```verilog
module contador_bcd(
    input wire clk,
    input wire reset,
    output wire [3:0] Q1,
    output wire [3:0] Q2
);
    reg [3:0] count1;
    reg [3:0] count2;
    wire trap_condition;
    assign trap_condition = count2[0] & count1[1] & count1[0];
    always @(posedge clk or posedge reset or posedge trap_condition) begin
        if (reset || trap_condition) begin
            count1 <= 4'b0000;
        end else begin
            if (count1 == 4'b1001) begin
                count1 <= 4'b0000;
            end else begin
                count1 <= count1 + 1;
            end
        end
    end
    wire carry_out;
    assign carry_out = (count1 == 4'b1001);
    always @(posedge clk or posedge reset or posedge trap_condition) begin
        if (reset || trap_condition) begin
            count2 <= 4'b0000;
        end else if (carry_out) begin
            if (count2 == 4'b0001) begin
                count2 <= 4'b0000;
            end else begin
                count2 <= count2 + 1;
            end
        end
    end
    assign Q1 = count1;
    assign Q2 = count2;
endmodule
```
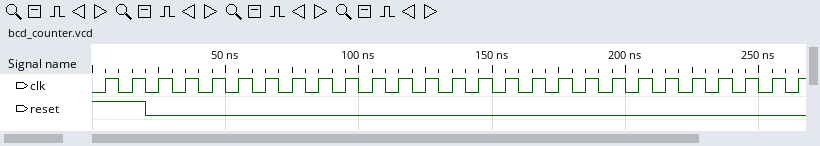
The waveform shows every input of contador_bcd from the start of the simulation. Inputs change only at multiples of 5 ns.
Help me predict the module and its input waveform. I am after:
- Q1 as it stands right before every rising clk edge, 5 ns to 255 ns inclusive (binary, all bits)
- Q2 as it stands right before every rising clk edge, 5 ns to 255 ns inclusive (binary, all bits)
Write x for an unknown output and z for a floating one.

0000, 0000, 0000, 0001, 0010, 0011, 0100, 0101, 0110, 0111, 1000, 1001, 0000, 0001, 0010, 0000, 0001, 0010, 0011, 0100, 0101, 0110, 0111, 1000, 1001, 0000
0000, 0000, 0000, 0000, 0000, 0000, 0000, 0000, 0000, 0000, 0000, 0000, 0001, 0001, 0001, 0000, 0000, 0000, 0000, 0000, 0000, 0000, 0000, 0000, 0000, 0001
